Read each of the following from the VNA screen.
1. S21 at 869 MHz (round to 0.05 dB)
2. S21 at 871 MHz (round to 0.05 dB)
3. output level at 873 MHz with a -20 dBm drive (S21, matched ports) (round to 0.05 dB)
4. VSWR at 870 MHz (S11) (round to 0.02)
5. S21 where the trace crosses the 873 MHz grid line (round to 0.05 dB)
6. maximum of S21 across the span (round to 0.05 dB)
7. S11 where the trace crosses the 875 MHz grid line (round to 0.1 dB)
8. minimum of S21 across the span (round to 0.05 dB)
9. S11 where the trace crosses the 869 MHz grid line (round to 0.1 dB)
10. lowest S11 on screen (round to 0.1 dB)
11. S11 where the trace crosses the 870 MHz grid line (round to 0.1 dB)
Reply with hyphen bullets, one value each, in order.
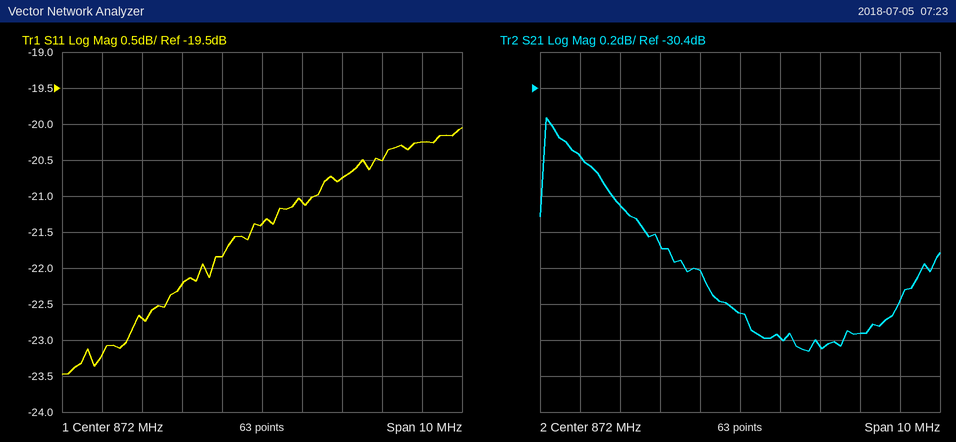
- -31.05 dB
- -31.40 dB
- -51.80 dBm
- 1.16
- -31.80 dB
- -30.55 dB
- -20.5 dB
- -31.85 dB
- -22.7 dB
- -23.5 dB
- -22.2 dB
